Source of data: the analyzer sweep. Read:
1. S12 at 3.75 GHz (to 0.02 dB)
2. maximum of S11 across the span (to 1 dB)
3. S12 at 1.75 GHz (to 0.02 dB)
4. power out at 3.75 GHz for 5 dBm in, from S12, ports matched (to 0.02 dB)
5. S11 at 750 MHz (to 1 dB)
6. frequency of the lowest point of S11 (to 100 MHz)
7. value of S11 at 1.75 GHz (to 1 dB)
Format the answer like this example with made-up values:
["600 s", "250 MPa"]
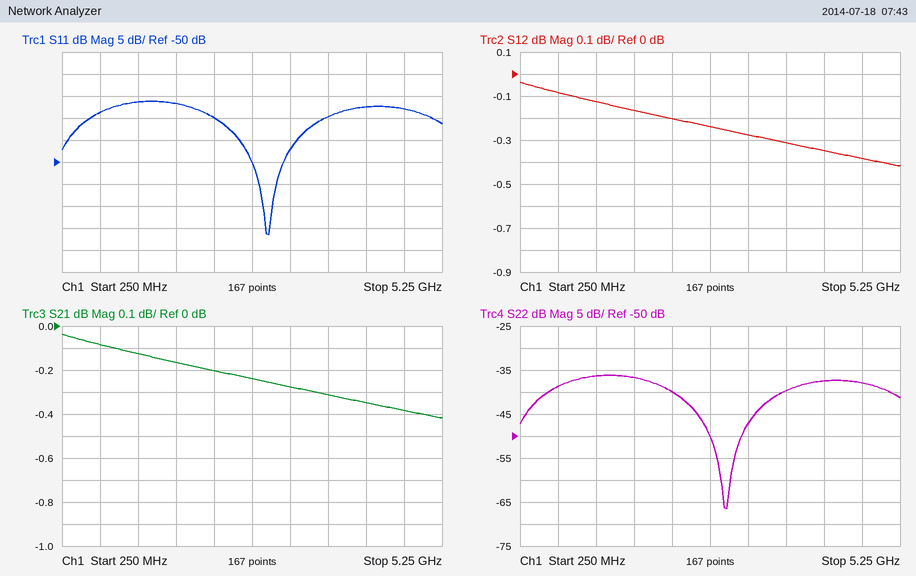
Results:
["-0.32 dB", "-36 dB", "-0.16 dB", "4.68 dBm", "-39 dB", "3.0 GHz", "-37 dB"]
